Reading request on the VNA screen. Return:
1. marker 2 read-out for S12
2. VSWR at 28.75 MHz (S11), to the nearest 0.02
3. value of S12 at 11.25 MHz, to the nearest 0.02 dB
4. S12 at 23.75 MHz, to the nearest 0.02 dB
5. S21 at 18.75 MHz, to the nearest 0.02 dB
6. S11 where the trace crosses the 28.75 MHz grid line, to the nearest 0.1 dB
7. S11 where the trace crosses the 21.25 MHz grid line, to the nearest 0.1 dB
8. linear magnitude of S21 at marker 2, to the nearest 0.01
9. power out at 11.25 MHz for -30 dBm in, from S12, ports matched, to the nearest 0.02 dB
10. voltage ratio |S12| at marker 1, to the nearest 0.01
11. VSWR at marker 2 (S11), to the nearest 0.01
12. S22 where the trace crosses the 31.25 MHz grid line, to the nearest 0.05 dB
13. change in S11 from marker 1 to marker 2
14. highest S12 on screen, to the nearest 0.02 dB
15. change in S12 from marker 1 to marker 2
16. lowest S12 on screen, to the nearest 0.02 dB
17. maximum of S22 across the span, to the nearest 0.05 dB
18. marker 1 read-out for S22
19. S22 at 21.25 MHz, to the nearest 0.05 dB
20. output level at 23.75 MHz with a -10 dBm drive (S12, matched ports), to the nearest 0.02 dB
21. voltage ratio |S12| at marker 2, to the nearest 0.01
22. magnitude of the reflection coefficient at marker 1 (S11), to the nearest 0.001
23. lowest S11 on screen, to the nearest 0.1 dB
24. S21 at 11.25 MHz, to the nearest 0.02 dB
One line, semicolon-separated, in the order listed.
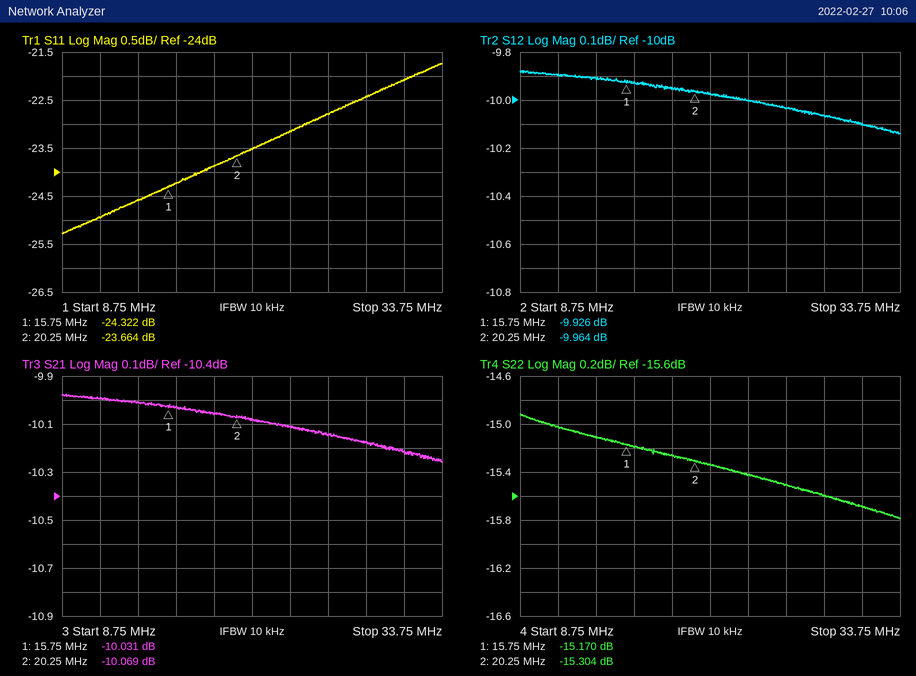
-9.964 dB; 1.16; -9.90 dB; -10.00 dB; -10.06 dB; -22.4 dB; -23.5 dB; 0.31; -39.90 dBm; 0.32; 1.14; -15.70 dB; 0.658 dB; -9.88 dB; -0.038 dB; -10.14 dB; -14.90 dB; -15.170 dB; -15.35 dB; -20.00 dBm; 0.32; 0.061; -25.3 dB; -10.00 dB
